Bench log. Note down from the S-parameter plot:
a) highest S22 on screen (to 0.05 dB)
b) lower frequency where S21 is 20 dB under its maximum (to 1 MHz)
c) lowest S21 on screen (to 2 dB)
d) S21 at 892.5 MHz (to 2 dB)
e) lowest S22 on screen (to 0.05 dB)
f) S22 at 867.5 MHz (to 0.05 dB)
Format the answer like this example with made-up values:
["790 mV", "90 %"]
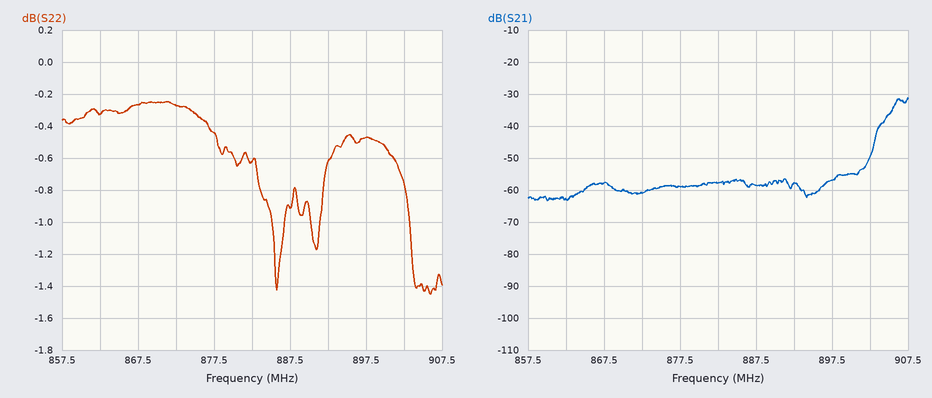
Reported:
["-0.25 dB", "902 MHz", "-64 dB", "-58 dB", "-1.45 dB", "-0.25 dB"]
